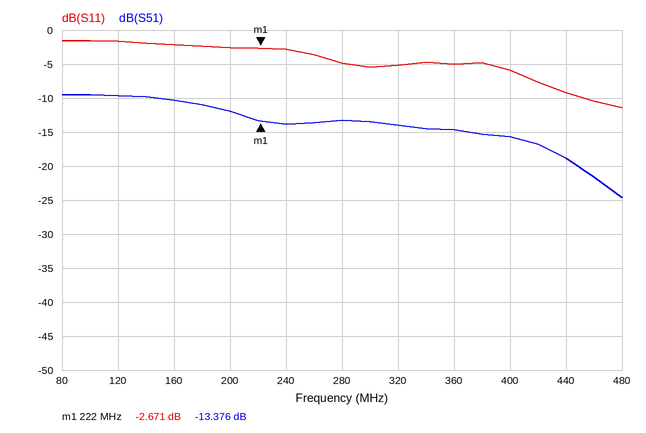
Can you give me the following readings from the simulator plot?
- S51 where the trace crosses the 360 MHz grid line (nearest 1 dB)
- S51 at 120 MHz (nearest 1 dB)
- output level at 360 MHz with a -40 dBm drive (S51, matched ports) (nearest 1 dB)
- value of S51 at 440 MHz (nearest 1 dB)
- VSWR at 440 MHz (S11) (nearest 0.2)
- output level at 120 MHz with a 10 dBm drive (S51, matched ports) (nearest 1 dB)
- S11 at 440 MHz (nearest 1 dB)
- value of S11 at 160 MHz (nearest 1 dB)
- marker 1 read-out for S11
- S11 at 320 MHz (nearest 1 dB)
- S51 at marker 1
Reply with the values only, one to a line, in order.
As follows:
-15 dB
-10 dB
-55 dBm
-19 dB
2.0
0 dBm
-9 dB
-2 dB
-2.671 dB
-5 dB
-13.376 dB
